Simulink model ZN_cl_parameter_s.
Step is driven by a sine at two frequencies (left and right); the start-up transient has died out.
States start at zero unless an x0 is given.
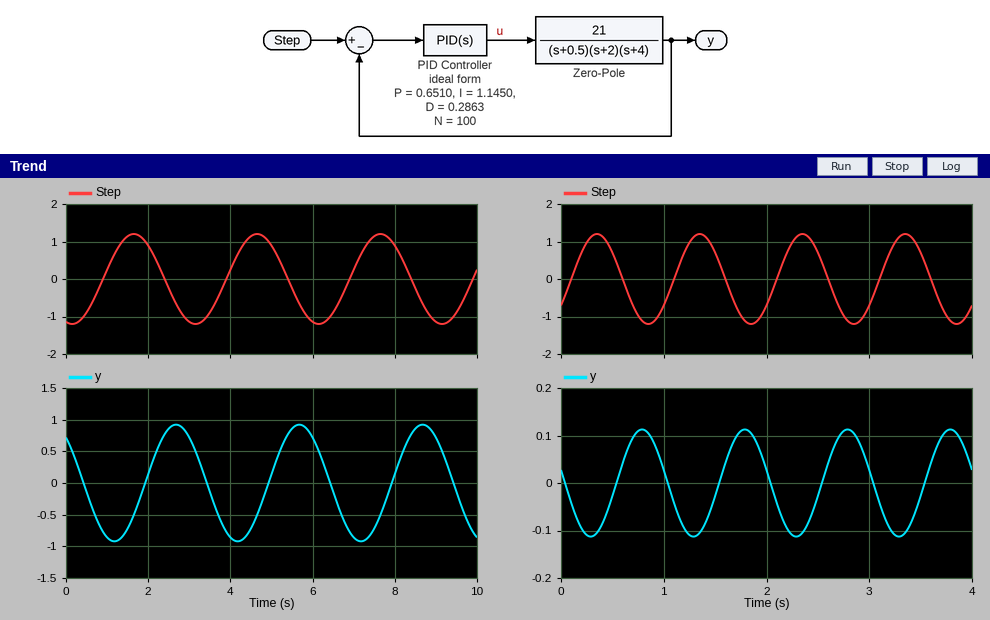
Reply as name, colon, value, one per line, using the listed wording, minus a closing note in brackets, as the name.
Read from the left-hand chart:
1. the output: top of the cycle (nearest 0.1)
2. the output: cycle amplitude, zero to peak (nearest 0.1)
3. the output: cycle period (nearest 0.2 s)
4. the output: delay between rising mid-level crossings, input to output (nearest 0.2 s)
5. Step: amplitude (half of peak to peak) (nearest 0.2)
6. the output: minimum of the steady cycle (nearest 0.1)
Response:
the output: top of the cycle: 0.9
the output: cycle amplitude, zero to peak: 0.9
the output: cycle period: 3.0 s
the output: delay between rising mid-level crossings, input to output: 1.0 s
Step: amplitude (half of peak to peak): 1.2
the output: minimum of the steady cycle: -0.9
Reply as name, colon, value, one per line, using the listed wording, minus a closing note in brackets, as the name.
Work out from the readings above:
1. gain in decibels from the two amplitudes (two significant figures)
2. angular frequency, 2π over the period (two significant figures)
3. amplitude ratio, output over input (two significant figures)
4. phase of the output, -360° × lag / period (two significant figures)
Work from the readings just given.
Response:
gain in decibels from the two amplitudes: -2.5 dB
angular frequency, 2π over the period: 2.1 rad/s
amplitude ratio, output over input: 0.75
phase of the output, -360° × lag / period: -120°
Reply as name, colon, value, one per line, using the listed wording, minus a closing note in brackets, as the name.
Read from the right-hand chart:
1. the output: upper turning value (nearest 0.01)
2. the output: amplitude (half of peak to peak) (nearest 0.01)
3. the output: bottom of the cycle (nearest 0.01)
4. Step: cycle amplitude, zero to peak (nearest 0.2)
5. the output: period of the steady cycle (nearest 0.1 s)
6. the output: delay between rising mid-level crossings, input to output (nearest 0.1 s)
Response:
the output: upper turning value: 0.11
the output: amplitude (half of peak to peak): 0.11
the output: bottom of the cycle: -0.11
Step: cycle amplitude, zero to peak: 1.2
the output: period of the steady cycle: 1.0 s
the output: delay between rising mid-level crossings, input to output: 0.4 s
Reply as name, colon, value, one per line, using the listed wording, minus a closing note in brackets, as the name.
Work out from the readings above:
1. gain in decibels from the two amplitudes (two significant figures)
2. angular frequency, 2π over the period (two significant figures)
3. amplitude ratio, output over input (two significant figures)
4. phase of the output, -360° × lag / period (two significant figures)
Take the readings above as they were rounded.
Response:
gain in decibels from the two amplitudes: -21 dB
angular frequency, 2π over the period: 6.3 rad/s
amplitude ratio, output over input: 0.092
phase of the output, -360° × lag / period: -140°
